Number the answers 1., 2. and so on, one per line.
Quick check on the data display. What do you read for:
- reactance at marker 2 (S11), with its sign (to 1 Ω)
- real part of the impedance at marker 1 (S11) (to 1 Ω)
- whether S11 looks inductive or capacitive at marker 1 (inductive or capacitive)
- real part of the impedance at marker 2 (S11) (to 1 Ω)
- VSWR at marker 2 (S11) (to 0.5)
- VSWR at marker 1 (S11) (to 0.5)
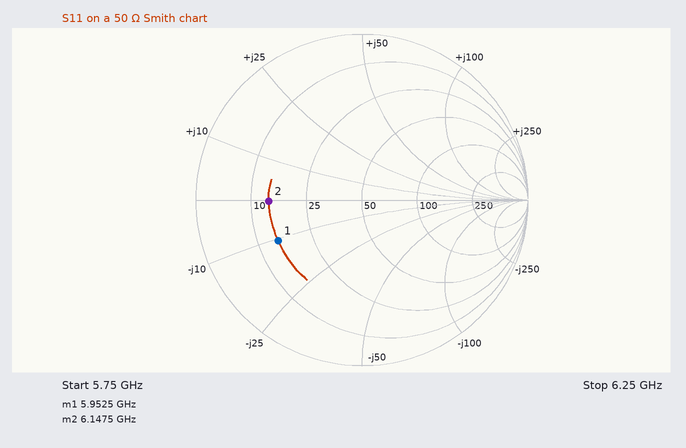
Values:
1. 0 Ω
2. 15 Ω
3. capacitive
4. 14 Ω
5. 3.5
6. 3.5
